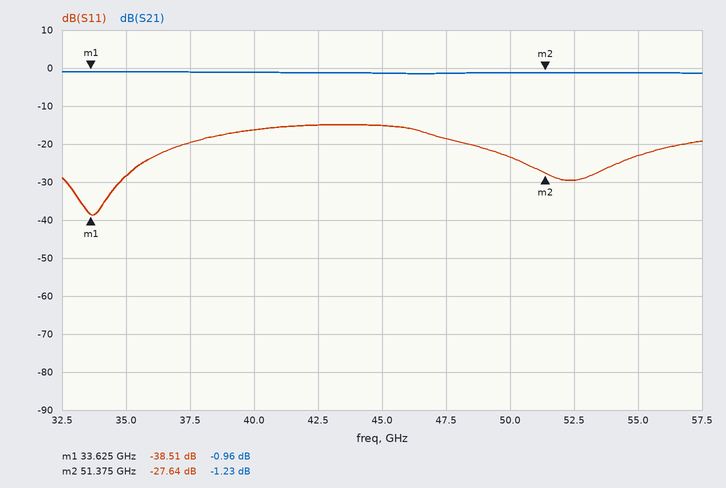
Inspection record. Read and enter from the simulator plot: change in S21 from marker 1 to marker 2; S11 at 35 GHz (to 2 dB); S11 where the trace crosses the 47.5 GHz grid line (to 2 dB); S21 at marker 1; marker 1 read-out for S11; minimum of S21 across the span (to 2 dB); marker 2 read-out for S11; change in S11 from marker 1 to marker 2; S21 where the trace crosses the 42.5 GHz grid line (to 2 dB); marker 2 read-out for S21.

-0.27 dB
-28 dB
-18 dB
-0.96 dB
-38.51 dB
-2 dB
-27.64 dB
10.87 dB
-2 dB
-1.23 dB
